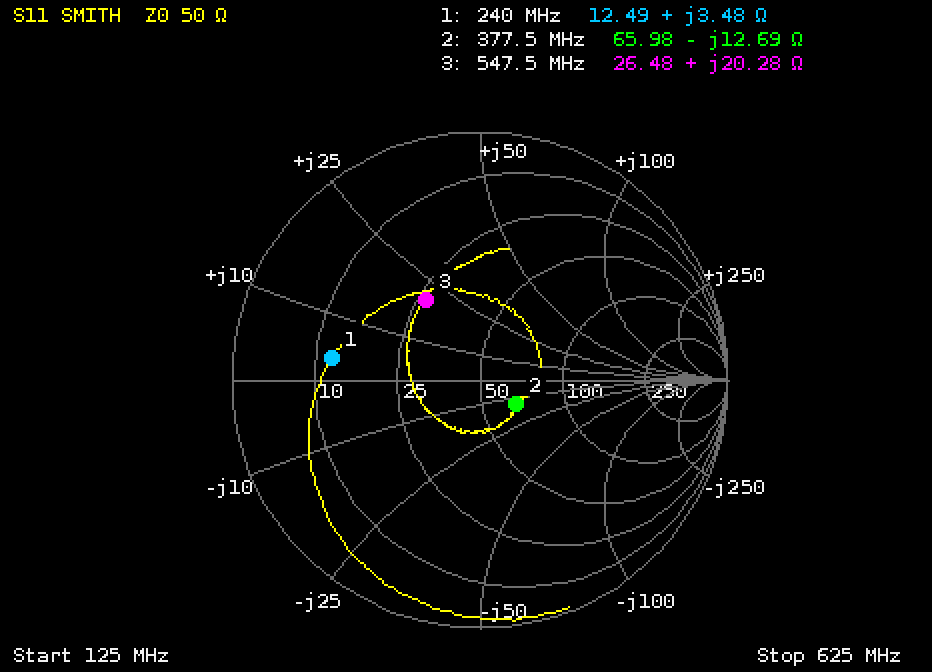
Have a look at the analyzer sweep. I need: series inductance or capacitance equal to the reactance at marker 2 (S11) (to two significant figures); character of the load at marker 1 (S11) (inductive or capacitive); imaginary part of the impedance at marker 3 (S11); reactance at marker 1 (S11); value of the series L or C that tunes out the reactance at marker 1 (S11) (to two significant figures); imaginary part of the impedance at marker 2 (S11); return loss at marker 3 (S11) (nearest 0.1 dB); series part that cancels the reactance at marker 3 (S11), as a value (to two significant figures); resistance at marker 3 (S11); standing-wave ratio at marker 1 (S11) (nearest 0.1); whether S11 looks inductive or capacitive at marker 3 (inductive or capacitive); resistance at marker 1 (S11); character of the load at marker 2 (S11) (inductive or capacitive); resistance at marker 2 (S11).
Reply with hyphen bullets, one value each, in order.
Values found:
- 33 pF
- inductive
- +20.28 Ω
- +3.48 Ω
- 190 pF
- -12.69 Ω
- 8.1 dB
- 14 pF
- 26.48 Ω
- 4.0
- inductive
- 12.49 Ω
- capacitive
- 65.98 Ω
